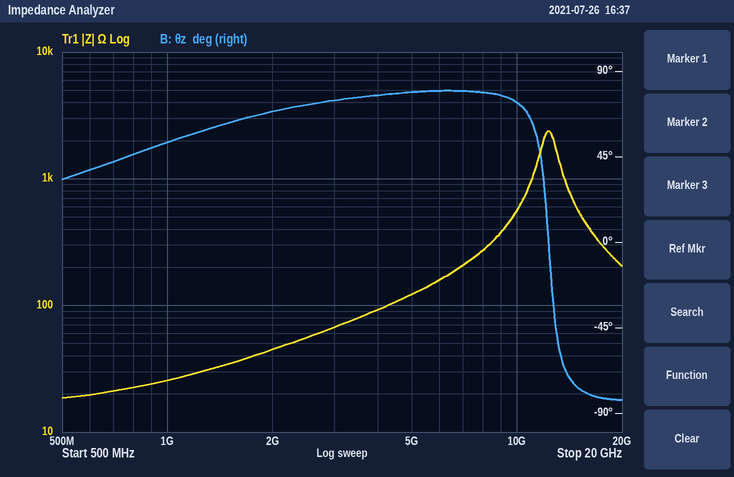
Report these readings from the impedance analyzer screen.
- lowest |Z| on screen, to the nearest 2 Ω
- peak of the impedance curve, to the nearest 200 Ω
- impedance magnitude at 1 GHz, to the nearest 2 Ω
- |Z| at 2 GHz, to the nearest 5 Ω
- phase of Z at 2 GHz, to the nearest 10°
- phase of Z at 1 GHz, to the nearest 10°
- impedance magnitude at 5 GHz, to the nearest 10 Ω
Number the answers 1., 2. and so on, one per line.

1. 18 Ω
2. 2.4 kΩ
3. 26 Ω
4. 45 Ω
5. 70°
6. 50°
7. 120 Ω
